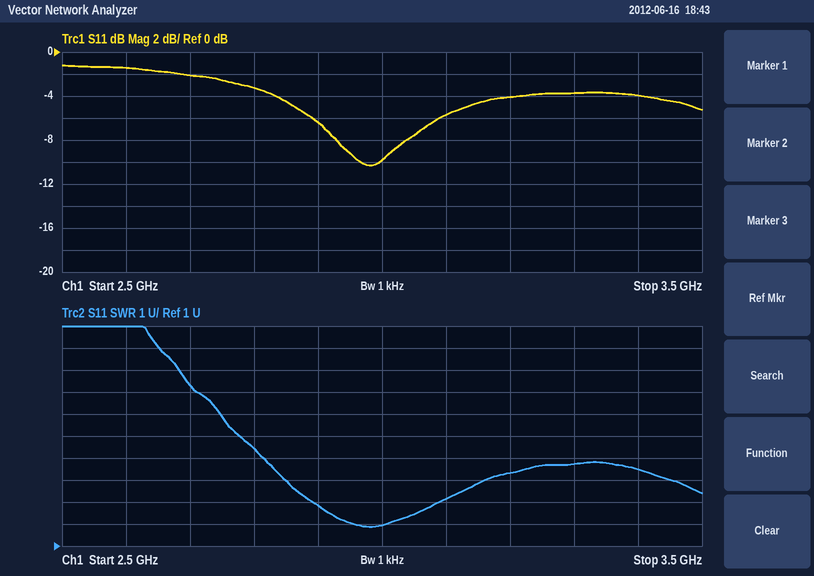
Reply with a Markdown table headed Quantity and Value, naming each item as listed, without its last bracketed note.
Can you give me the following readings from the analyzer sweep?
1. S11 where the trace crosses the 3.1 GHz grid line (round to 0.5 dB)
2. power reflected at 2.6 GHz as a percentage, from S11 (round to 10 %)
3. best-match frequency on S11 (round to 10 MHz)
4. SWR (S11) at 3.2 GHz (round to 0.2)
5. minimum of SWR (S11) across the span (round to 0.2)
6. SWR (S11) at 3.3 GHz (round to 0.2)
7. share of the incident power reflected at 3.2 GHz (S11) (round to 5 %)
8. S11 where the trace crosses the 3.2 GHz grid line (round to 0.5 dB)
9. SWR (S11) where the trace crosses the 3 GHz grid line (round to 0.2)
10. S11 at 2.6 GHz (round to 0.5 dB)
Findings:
| Quantity | Value |
|---|---|
| S11 where the trace crosses the 3.1 GHz grid line | -5.5 dB |
| power reflected at 2.6 GHz as a percentage, from S11 | 70 % |
| best-match frequency on S11 | 2.98 GHz |
| SWR (S11) at 3.2 GHz | 4.4 |
| minimum of SWR (S11) across the span | 1.8 |
| SWR (S11) at 3.3 GHz | 4.8 |
| share of the incident power reflected at 3.2 GHz (S11) | 40 % |
| S11 where the trace crosses the 3.2 GHz grid line | -4.0 dB |
| SWR (S11) where the trace crosses the 3 GHz grid line | 2.0 |
| S11 at 2.6 GHz | -1.5 dB |
